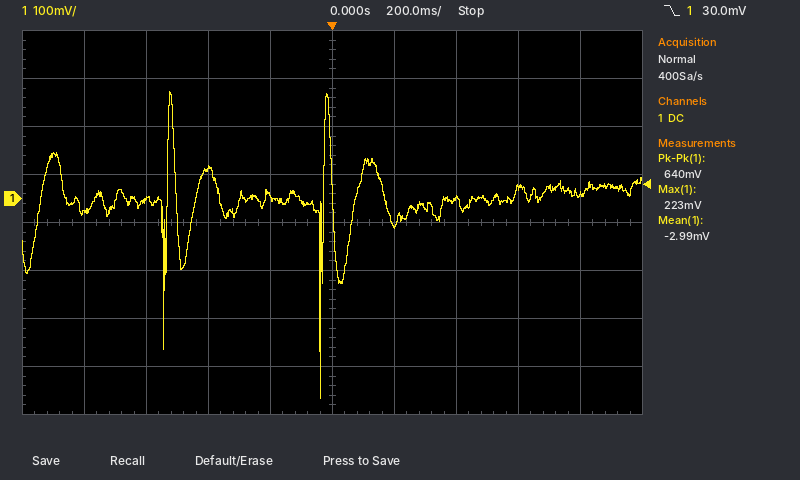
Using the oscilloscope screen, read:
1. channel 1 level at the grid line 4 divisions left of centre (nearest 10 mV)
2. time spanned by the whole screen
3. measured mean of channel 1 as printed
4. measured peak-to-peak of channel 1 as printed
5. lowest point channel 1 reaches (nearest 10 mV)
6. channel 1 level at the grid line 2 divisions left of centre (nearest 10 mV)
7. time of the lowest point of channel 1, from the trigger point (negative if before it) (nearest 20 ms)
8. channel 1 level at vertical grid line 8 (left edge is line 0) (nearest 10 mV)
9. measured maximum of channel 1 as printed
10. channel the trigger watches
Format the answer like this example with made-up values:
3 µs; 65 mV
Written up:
-30 mV; 2 s; -2.99 mV; 640 mV; -420 mV; 60 mV; -40 ms; 20 mV; 223 mV; channel 1
